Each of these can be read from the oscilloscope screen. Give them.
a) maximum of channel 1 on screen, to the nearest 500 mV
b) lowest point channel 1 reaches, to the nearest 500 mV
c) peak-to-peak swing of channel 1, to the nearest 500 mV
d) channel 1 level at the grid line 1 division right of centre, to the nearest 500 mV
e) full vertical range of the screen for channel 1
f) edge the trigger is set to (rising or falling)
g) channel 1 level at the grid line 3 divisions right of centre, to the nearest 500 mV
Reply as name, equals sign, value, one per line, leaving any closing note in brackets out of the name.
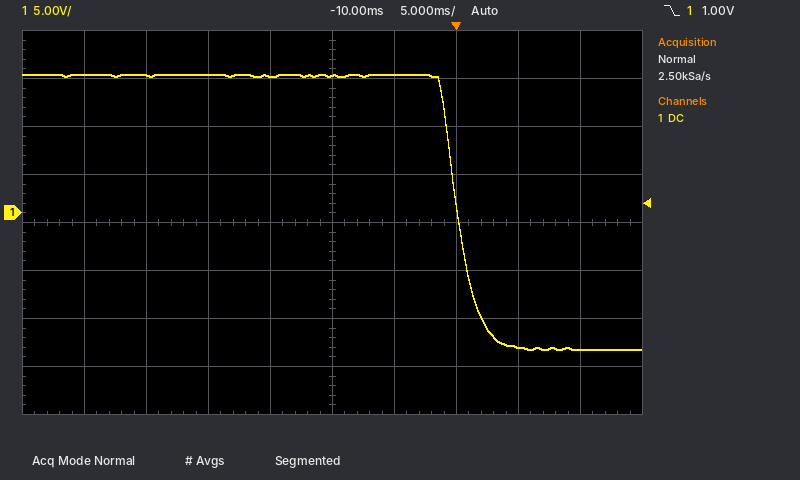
maximum of channel 1 on screen, to the nearest 500 mV = 14.5 V
lowest point channel 1 reaches, to the nearest 500 mV = -14.0 V
peak-to-peak swing of channel 1, to the nearest 500 mV = 28.5 V
channel 1 level at the grid line 1 division right of centre, to the nearest 500 mV = 14.5 V
full vertical range of the screen for channel 1 = 40 V
edge the trigger is set to = falling
channel 1 level at the grid line 3 divisions right of centre, to the nearest 500 mV = -14.0 V
